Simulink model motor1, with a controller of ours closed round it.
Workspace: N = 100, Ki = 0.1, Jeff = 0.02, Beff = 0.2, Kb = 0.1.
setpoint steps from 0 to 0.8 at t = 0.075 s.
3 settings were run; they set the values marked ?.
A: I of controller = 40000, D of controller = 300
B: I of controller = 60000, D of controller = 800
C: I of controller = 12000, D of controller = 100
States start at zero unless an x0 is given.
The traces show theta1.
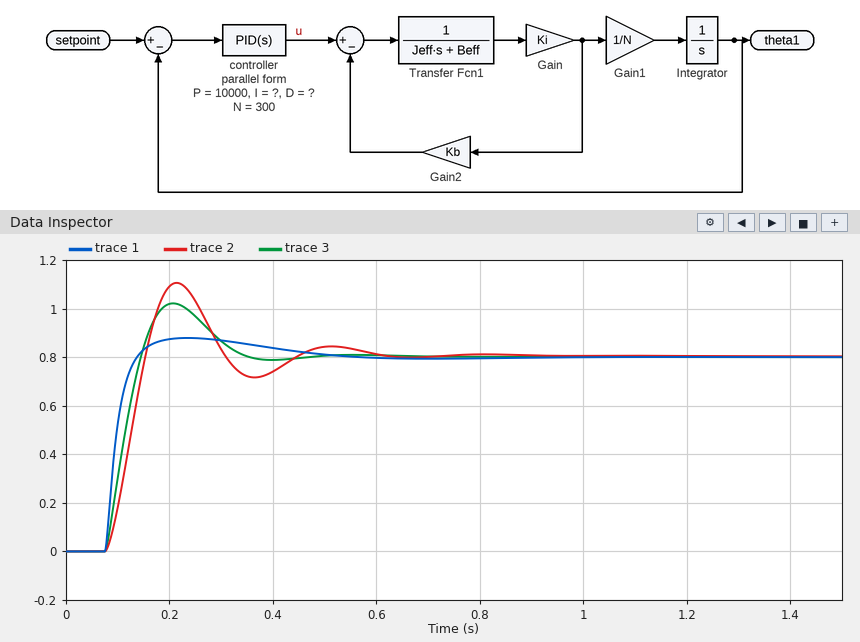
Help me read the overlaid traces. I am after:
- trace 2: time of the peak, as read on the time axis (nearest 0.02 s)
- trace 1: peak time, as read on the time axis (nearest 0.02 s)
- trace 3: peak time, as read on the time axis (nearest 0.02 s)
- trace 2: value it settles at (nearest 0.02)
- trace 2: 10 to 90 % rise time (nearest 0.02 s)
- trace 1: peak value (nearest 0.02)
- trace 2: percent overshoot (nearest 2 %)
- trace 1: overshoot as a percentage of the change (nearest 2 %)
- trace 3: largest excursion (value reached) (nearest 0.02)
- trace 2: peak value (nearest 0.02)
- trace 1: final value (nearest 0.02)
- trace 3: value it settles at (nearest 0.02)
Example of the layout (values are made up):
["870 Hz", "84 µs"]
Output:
["0.22 s", "0.24 s", "0.20 s", "0.80", "0.06 s", "0.88", "38 %", "10 %", "1.02", "1.10", "0.80", "0.80"]
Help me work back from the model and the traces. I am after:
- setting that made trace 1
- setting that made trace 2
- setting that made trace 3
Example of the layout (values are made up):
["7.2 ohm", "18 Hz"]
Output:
["B", "C", "A"]
